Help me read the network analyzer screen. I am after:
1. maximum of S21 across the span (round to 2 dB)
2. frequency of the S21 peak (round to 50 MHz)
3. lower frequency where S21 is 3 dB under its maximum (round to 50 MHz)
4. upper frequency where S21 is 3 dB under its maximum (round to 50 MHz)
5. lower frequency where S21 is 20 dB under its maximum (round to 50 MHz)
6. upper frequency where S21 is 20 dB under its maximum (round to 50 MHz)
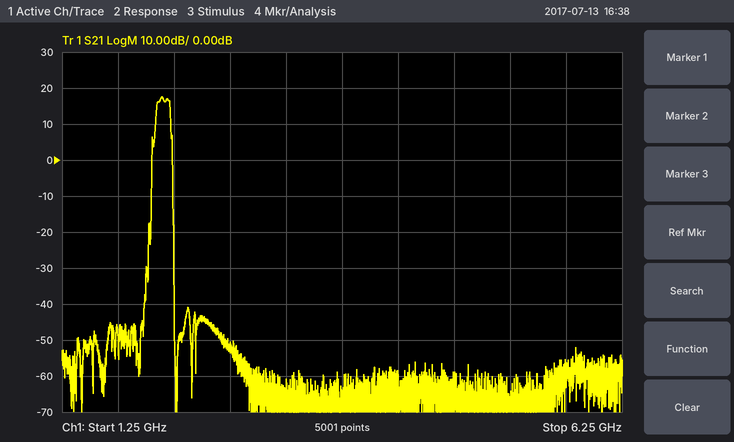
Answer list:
18 dB
2.15 GHz
2.10 GHz
2.20 GHz
2.05 GHz
2.25 GHz
